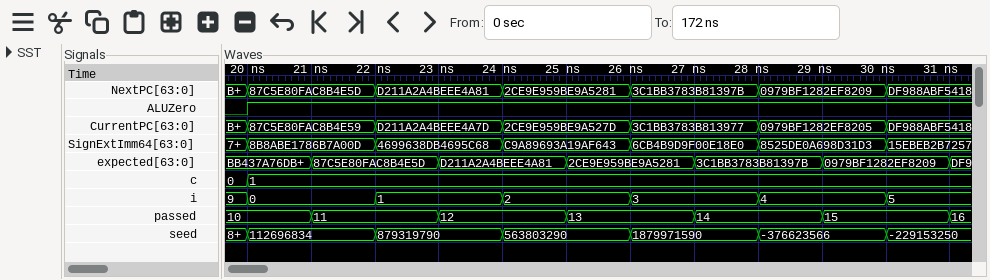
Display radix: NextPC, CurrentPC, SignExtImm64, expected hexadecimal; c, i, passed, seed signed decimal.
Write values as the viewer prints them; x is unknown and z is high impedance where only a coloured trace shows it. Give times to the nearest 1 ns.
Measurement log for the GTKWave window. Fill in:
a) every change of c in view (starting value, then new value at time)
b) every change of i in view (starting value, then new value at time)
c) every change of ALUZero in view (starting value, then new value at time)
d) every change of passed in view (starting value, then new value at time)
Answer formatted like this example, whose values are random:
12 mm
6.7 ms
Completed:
0, 1 at 20 ns
9, 0 at 20 ns, 1 at 22 ns, 2 at 24 ns, 3 at 26 ns, 4 at 28 ns, 5 at 30 ns
0, 1 at 20 ns
10, 11 at 21 ns, 12 at 23 ns, 13 at 25 ns, 14 at 27 ns, 15 at 29 ns, 16 at 31 ns
